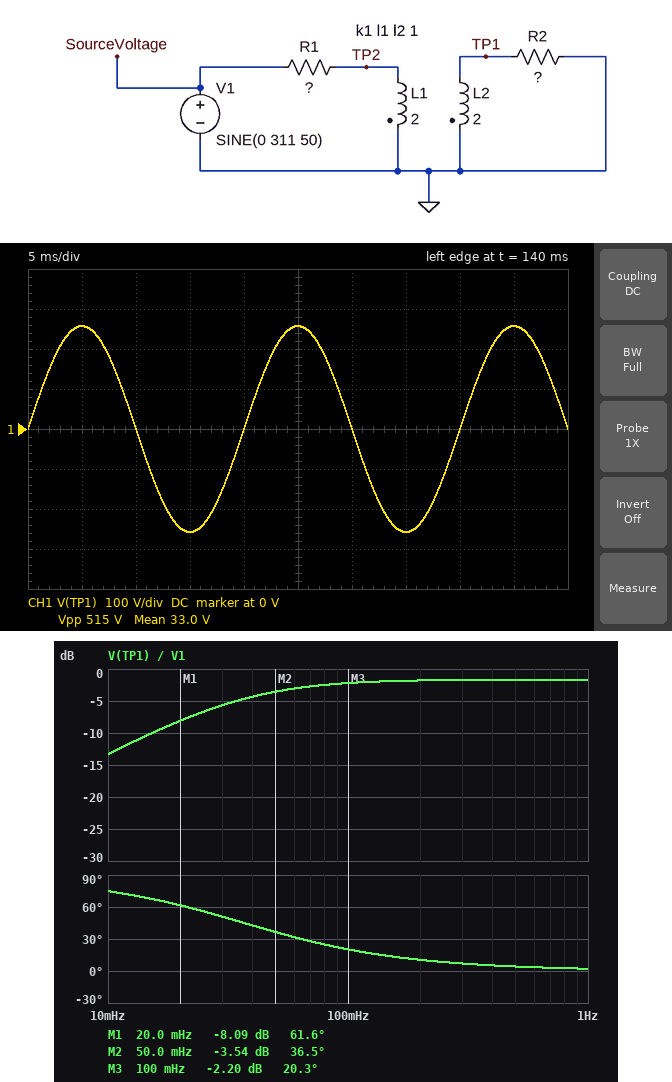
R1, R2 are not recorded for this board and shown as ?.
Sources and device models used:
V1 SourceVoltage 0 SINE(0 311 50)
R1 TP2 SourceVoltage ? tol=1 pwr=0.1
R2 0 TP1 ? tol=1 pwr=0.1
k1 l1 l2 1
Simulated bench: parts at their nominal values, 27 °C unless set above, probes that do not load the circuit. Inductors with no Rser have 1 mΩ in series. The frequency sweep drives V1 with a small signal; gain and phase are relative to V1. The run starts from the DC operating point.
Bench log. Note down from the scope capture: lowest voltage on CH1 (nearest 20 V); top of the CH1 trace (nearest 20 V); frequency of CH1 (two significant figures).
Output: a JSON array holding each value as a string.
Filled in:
["-260 V", "260 V", "50 Hz"]
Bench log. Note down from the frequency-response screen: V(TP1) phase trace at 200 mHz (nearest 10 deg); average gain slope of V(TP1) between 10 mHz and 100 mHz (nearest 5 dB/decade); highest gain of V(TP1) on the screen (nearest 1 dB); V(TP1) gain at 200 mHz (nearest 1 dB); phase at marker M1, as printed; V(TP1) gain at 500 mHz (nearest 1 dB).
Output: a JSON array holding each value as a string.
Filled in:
["10 deg", "10 dB/decade", "-2 dB", "-2 dB", "61.6 deg", "-2 dB"]
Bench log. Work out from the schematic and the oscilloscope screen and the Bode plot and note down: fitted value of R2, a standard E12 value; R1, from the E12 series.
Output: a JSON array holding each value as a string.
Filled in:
["2.7 Ω", "0.56 Ω"]
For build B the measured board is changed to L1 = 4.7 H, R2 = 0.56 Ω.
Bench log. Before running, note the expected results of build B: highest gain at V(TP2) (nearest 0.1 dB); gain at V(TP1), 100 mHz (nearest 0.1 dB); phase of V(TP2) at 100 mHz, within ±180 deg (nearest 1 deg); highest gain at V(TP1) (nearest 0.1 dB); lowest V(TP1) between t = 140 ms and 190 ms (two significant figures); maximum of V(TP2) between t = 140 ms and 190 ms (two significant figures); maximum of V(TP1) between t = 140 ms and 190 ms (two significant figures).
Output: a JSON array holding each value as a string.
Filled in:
["-3.1 dB", "-6.9 dB", "8 deg", "-6.8 dB", "-140 V", "220 V", "140 V"]
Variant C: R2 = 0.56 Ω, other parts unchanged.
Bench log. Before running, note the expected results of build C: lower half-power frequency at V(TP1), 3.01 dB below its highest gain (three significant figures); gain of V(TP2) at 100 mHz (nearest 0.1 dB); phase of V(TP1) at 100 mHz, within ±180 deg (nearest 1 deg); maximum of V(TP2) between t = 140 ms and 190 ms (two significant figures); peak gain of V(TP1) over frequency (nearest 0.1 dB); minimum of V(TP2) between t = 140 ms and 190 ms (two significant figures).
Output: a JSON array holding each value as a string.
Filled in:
["22.3 mHz", "-6.2 dB", "13 deg", "160 V", "-6.0 dB", "-160 V"]
